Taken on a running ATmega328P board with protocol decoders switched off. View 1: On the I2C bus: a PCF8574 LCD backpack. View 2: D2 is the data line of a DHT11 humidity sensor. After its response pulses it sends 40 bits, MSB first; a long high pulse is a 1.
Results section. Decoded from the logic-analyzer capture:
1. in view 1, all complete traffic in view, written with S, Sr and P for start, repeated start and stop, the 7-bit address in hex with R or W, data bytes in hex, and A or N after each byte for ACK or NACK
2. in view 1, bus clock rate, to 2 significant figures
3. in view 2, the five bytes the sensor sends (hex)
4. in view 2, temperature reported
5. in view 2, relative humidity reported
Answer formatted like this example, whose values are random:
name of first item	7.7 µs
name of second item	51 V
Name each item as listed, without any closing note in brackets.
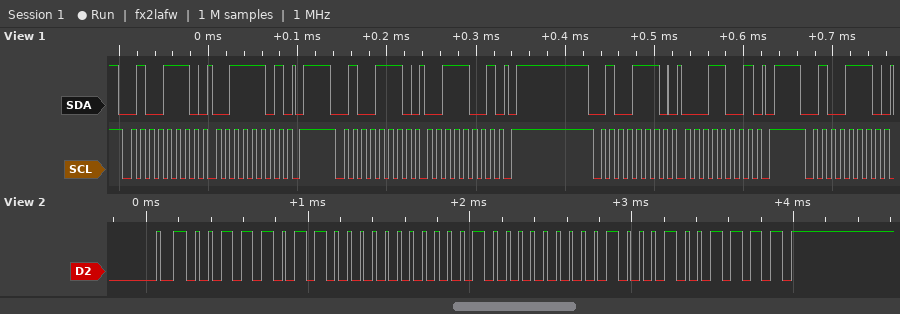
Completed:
in view 1, all complete traffic in view, written with S, Sr and P for start, repeated start and stop, the 7-bit address in hex with R or W, data bytes in hex, and A or N after each byte for ACK or NACK	S 27W A 3D A P S 27W A 39 A P S 27W A 19 A P S 27W A
in view 1, bus clock rate, to 2 significant figures	100 kHz
in view 2, the five bytes the sensor sends	3B 00 10 04 4F
in view 2, temperature reported	16.4 °C
in view 2, relative humidity reported	59 %
